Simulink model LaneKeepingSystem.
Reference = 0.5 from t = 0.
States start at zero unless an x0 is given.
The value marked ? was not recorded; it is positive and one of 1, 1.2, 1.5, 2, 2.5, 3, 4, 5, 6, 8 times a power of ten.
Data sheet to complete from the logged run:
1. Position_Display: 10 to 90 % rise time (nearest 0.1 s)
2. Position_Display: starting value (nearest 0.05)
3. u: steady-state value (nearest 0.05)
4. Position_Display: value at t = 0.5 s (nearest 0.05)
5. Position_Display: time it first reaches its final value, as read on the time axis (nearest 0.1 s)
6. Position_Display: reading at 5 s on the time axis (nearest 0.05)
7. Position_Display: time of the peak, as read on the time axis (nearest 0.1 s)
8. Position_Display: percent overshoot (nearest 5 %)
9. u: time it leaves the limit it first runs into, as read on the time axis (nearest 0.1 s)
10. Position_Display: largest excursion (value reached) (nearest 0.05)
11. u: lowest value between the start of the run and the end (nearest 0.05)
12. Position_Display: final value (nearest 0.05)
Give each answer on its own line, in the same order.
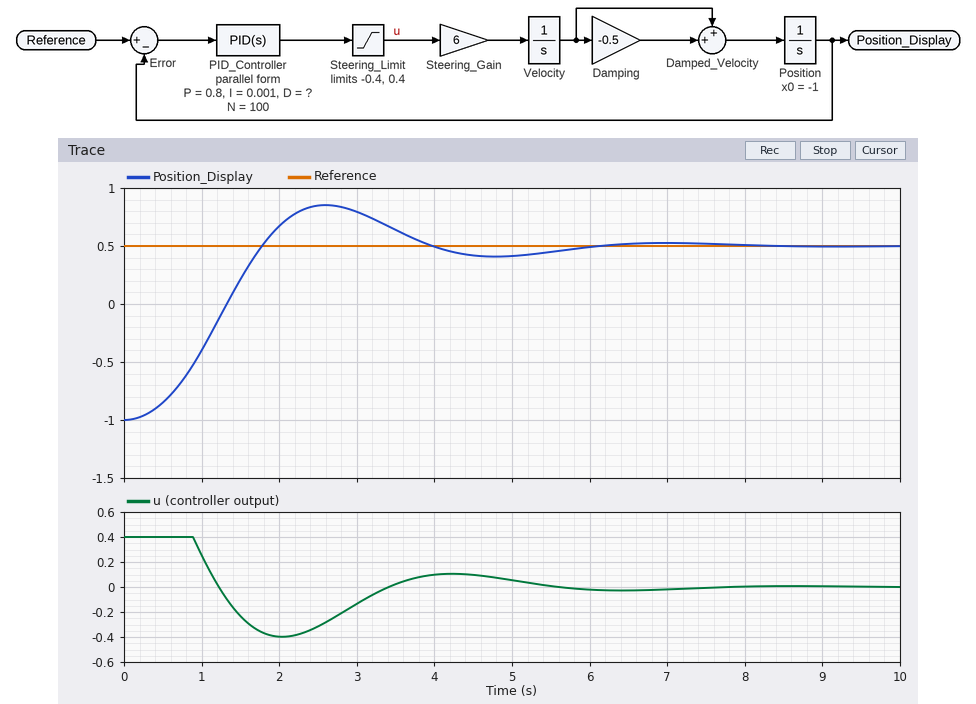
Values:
1.1 s
-1.00
0.00
-0.85
1.8 s
0.40
2.6 s
25 %
0.9 s
0.85
-0.40
0.50
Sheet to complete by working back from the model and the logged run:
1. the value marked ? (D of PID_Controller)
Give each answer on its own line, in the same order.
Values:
0.4
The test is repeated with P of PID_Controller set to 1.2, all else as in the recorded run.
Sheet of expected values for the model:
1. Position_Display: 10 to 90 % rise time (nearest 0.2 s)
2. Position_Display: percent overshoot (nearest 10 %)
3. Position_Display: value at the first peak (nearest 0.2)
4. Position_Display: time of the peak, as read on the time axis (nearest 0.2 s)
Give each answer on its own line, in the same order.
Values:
1.0 s
40 %
1.0
2.6 s
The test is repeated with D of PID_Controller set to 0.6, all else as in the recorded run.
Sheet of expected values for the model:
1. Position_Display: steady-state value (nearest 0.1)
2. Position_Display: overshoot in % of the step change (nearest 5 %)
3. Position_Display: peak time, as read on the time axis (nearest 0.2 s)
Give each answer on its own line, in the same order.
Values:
0.5
10 %
2.8 s
